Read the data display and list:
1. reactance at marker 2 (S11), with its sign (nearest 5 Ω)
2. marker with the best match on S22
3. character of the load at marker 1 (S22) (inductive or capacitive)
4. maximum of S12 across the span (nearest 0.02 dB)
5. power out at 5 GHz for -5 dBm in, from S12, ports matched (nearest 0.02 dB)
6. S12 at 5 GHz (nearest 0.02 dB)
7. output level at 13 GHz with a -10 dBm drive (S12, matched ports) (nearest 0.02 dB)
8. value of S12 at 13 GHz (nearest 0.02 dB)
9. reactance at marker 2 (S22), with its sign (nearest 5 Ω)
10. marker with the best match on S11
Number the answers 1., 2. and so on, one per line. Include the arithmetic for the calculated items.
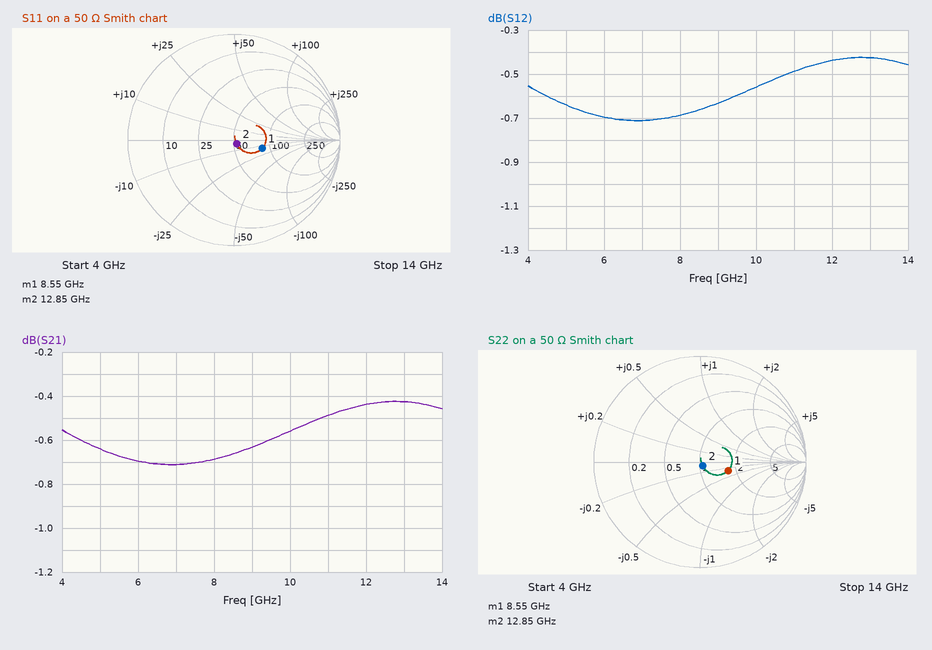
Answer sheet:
1. -5 Ω
2. marker 2
3. capacitive
4. -0.42 dB
5. -5 dBm + (-0.64 dB) = -5.64 dBm
6. -0.64 dB
7. -10 dBm + (-0.42 dB) = -10.42 dBm
8. -0.42 dB
9. -5 Ω
10. marker 2
